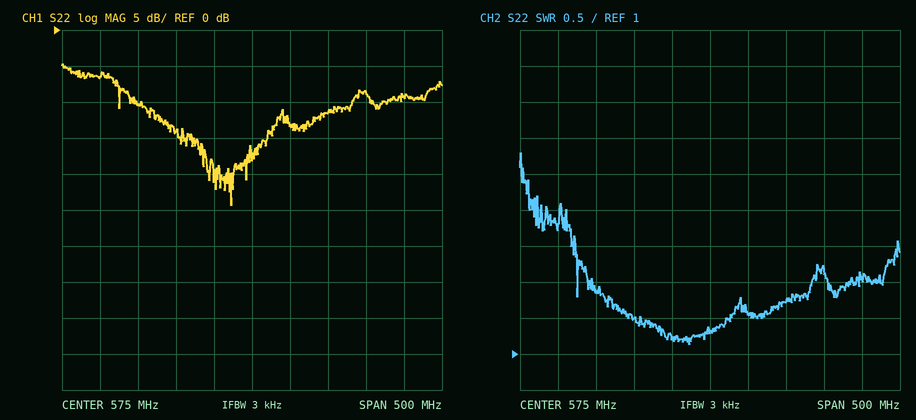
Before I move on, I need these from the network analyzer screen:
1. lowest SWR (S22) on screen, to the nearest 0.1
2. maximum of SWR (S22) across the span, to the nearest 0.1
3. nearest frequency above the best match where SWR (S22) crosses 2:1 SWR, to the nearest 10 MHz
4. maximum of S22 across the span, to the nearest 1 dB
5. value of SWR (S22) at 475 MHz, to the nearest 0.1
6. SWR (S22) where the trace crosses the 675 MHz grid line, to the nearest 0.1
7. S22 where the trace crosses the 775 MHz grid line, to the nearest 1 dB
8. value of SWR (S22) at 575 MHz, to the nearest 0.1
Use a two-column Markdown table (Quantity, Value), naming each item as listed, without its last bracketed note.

| Quantity | Value |
|---|---|
| lowest SWR (S22) on screen, to the nearest 0.1 | 1.1 |
| maximum of SWR (S22) across the span, to the nearest 0.1 | 3.8 |
| nearest frequency above the best match where SWR (S22) crosses 2:1 SWR, to the nearest 10 MHz | 710 MHz |
| maximum of S22 across the span, to the nearest 1 dB | -5 dB |
| value of SWR (S22) at 475 MHz, to the nearest 0.1 | 1.5 |
| SWR (S22) where the trace crosses the 675 MHz grid line, to the nearest 0.1 | 1.7 |
| S22 where the trace crosses the 775 MHz grid line, to the nearest 1 dB | -9 dB |
| value of SWR (S22) at 575 MHz, to the nearest 0.1 | 1.3 |
